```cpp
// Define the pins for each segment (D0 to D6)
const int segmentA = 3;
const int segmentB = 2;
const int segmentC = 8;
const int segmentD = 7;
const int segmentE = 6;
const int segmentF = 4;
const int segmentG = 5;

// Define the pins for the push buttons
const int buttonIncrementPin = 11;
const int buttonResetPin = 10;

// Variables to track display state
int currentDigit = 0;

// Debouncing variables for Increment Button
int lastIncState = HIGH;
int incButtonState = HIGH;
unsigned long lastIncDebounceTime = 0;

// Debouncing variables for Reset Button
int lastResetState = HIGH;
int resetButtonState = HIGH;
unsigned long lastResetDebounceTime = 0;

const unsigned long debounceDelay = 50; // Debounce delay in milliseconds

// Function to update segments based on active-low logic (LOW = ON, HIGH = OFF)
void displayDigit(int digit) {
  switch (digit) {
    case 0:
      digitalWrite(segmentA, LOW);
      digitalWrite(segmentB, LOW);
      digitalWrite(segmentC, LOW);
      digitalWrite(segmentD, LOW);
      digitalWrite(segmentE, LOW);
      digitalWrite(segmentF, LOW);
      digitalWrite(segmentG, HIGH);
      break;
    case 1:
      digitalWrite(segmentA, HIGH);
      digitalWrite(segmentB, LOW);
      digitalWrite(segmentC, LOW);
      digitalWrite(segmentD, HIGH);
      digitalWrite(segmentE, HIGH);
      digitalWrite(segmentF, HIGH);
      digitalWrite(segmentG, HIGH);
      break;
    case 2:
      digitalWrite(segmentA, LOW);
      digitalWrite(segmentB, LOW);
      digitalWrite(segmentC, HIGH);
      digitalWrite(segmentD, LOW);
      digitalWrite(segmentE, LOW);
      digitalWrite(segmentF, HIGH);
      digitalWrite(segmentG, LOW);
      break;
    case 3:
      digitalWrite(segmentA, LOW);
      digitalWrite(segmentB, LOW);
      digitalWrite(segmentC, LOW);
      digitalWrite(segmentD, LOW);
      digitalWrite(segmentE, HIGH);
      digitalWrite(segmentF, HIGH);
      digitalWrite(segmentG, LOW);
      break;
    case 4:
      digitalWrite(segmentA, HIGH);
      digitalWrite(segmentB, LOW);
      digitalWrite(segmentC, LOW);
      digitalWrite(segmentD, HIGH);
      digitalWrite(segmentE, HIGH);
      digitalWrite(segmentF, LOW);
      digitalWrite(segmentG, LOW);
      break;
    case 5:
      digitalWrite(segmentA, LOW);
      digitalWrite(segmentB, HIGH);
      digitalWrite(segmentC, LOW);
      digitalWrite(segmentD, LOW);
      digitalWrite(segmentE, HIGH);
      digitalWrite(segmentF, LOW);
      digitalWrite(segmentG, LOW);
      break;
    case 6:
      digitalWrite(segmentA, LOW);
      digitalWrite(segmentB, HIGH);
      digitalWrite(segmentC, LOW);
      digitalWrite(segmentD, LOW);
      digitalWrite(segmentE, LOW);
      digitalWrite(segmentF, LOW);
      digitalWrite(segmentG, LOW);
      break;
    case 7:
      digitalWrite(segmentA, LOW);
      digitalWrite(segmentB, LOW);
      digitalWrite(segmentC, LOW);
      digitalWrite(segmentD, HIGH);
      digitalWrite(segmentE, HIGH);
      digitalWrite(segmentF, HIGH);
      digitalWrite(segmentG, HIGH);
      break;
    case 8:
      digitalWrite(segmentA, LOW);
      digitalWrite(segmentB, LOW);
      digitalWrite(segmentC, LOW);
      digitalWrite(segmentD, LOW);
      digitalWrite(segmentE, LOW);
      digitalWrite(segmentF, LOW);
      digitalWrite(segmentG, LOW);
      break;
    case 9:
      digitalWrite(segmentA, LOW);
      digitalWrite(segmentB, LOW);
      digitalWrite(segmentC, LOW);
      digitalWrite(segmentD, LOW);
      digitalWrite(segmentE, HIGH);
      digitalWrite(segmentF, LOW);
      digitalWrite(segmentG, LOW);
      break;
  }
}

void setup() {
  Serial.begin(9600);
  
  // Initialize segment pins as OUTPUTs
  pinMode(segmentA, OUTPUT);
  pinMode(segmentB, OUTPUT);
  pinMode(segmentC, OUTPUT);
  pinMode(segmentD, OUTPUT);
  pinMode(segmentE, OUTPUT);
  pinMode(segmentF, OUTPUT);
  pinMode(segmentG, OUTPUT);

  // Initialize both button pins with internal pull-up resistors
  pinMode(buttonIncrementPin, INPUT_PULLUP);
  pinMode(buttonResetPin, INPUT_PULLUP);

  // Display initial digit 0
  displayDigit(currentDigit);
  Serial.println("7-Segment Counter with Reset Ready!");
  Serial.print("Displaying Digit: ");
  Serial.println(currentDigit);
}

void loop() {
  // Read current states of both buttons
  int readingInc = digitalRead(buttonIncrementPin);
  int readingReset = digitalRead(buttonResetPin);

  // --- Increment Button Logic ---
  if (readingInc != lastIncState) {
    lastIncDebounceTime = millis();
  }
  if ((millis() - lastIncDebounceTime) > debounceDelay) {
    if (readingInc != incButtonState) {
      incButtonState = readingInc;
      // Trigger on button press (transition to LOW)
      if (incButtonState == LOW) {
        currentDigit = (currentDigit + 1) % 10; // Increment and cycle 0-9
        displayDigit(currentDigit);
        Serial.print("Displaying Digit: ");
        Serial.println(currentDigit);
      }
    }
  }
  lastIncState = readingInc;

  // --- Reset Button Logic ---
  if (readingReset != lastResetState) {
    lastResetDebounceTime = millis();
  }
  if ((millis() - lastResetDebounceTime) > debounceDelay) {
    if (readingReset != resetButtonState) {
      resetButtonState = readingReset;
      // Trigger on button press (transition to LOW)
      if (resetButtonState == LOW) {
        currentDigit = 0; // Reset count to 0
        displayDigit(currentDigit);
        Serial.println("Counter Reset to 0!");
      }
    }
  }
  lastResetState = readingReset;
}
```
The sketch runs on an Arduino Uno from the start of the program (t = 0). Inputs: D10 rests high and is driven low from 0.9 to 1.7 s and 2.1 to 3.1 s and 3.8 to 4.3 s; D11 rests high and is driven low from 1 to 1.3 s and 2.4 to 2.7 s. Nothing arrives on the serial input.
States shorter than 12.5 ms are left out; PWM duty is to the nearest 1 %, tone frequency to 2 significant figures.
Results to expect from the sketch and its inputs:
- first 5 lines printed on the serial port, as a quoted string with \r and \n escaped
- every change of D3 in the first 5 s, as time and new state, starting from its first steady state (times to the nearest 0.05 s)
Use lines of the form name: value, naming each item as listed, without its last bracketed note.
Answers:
first 5 lines printed on the serial port, as a quoted string with \r and \n escaped: "7-Segment Counter with Reset Ready!\r\nDisplaying Digit: 0\r\nCounter Reset to 0!\r\nDisplaying Digit: 1\r\nCounter Reset to 0!\r\n"
every change of D3 in the first 5 s, as time and new state, starting from its first steady state: 0 s low; 1.05 s high; 2.15 s low; 2.45 s high; 3.85 s low
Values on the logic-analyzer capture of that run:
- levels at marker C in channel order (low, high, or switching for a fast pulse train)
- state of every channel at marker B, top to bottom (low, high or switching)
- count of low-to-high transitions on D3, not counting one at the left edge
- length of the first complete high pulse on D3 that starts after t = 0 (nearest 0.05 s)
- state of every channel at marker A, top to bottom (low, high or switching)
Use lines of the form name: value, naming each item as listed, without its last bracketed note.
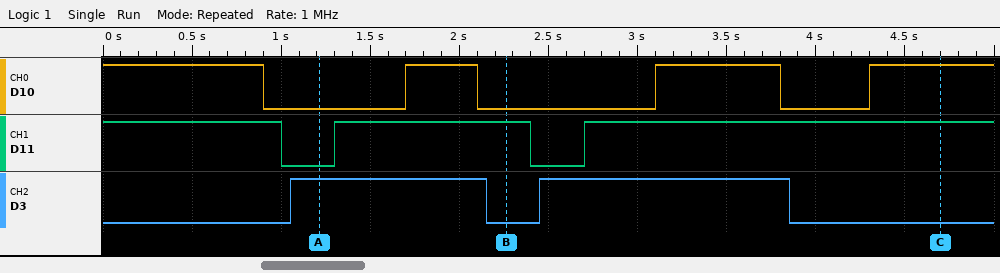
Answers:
levels at marker C in channel order: D10 high, D11 high, D3 low
state of every channel at marker B, top to bottom: D10 low, D11 high, D3 low
count of low-to-high transitions on D3, not counting one at the left edge: 2
length of the first complete high pulse on D3 that starts after t = 0: 1.10 s
state of every channel at marker A, top to bottom: D10 low, D11 low, D3 high
